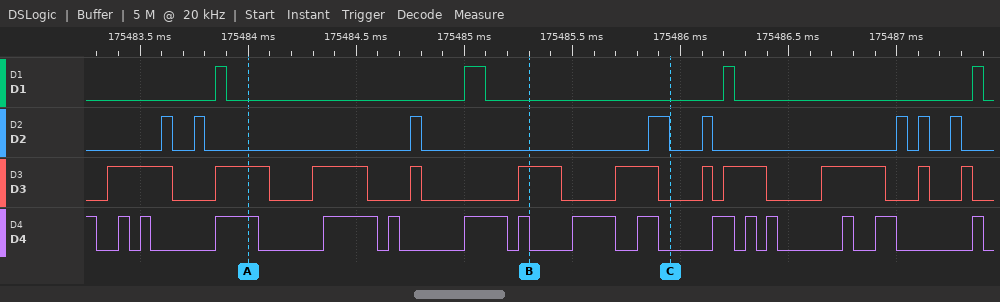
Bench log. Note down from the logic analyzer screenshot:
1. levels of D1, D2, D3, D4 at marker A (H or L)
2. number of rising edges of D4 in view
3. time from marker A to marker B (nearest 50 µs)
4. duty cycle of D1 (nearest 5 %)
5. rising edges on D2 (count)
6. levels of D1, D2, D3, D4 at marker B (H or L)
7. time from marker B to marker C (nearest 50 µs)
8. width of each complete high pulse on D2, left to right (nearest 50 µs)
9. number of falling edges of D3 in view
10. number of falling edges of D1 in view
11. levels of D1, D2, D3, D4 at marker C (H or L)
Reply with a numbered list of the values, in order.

1. D1=L, D2=L, D3=H, D4=H
2. 15
3. 1300 µs
4. 5 %
5. 8
6. D1=L, D2=L, D3=H, D4=L
7. 650 µs
8. 50 µs, 50 µs, 50 µs, 100 µs, 50 µs, 50 µs, 50 µs, 50 µs
9. 11
10. 4
11. D1=L, D2=L, D3=L, D4=L
